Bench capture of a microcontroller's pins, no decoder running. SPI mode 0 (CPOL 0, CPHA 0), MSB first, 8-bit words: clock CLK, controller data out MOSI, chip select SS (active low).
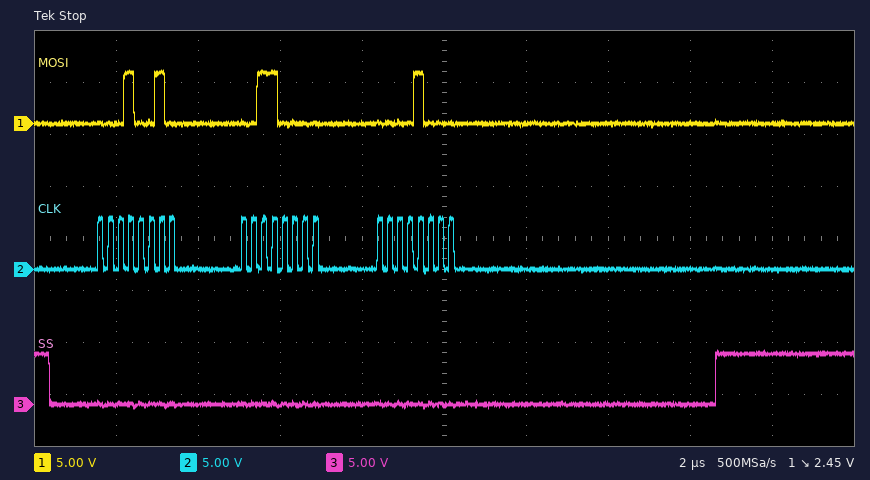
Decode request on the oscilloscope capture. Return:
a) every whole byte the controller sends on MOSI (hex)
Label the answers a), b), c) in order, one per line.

a) 12 30 08
